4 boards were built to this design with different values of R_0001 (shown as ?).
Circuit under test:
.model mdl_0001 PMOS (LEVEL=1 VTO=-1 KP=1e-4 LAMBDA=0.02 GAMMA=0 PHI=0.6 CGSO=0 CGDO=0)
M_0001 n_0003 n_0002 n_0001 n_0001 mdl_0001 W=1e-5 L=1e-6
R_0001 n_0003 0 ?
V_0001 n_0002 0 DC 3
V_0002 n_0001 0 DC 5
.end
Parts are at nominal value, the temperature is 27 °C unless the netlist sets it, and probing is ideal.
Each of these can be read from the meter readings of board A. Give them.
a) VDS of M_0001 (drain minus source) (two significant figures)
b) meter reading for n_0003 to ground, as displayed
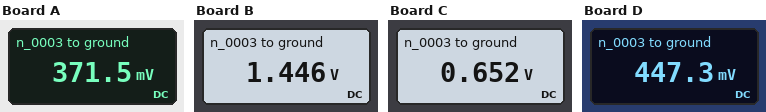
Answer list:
-4.6 V
371.5 mV
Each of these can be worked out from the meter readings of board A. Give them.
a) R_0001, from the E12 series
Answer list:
680 Ω
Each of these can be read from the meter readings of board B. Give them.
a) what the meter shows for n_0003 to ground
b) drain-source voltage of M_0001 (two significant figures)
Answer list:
1.446 V
-3.6 V
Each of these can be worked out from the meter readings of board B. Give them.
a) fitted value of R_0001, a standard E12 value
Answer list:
2.7 kΩ
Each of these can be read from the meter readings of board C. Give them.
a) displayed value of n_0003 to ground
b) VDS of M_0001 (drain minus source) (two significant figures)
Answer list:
0.652 V
-4.3 V
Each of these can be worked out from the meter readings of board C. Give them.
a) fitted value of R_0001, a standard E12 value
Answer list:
1.2 kΩ
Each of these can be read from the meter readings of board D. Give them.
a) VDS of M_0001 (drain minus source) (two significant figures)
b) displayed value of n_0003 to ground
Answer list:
-4.6 V
447.3 mV
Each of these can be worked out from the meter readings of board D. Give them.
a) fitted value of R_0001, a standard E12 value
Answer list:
820 Ω
